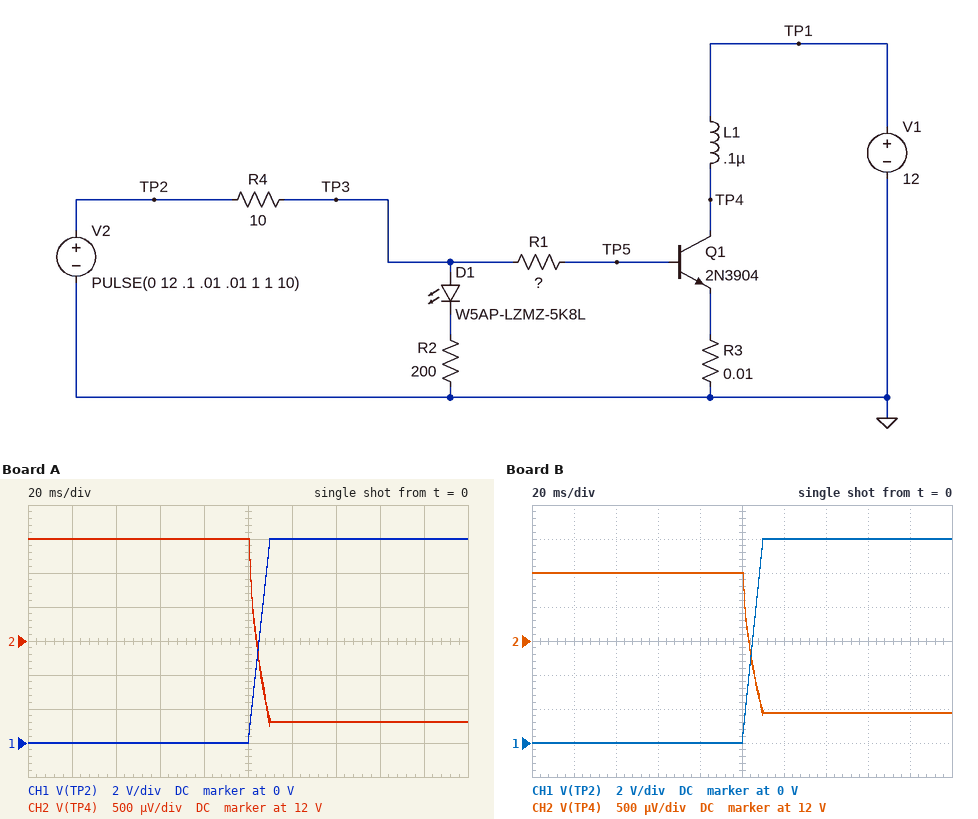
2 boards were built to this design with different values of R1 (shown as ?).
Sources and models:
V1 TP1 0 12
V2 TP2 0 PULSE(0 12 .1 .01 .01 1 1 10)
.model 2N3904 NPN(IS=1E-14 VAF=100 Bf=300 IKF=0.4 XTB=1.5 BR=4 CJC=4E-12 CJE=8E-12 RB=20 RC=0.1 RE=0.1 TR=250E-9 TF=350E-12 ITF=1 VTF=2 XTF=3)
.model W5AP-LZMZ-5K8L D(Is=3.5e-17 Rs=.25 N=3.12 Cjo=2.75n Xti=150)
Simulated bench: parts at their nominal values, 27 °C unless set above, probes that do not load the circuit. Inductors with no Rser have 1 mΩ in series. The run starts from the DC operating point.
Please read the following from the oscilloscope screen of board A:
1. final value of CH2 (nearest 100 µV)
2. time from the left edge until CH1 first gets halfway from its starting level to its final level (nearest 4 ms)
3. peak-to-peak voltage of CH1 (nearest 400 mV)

11.9973 V
104 ms
12.0 V
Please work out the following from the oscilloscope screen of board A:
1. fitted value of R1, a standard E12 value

150 Ω
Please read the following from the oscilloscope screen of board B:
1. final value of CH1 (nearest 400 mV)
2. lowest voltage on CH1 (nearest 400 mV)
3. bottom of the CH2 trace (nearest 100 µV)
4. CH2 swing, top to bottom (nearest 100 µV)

12.0 V
0 V
11.9979 V
2.1 mV
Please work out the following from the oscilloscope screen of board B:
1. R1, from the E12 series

270 Ω
